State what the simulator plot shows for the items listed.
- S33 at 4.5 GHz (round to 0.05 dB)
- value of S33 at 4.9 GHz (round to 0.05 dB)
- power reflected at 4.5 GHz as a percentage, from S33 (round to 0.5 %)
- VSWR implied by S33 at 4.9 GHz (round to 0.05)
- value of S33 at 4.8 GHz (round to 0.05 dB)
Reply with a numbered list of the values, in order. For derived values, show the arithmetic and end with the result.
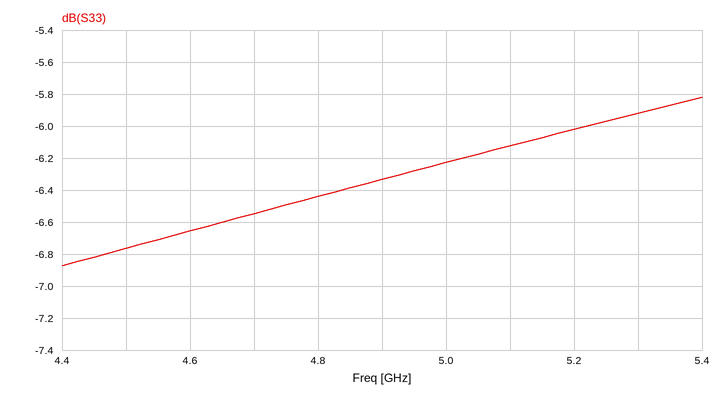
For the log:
1. -6.75 dB
2. -6.35 dB
3. 10^(-6.75/10) ≈ 21.1 %, so 21.0 % to the nearest 0.5 %
4. |Γ| = 10^(-6.35/20) = 0.4814; VSWR = (1 + 0.4814)/(1 − 0.4814) ≈ 2.86, so 2.85 to the nearest 0.05
5. -6.45 dB
